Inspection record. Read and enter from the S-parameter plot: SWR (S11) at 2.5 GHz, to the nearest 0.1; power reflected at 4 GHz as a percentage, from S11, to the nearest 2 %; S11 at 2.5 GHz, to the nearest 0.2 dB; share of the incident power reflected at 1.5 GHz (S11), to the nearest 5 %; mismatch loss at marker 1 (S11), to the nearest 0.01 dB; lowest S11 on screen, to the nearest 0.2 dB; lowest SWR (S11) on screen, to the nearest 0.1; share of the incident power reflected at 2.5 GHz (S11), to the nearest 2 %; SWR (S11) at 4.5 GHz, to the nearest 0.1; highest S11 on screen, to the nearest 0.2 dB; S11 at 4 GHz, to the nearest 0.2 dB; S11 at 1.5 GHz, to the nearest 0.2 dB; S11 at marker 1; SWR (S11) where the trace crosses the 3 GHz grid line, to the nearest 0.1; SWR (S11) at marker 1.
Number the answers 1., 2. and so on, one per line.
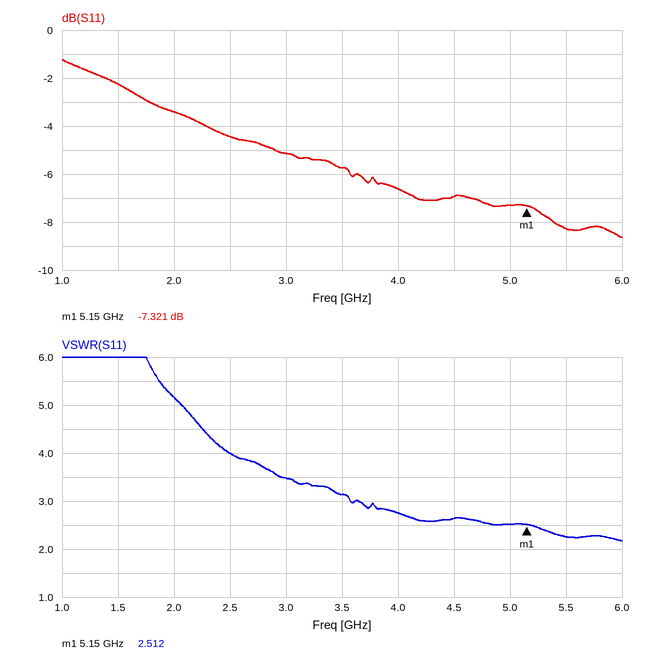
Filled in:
1. 4.0
2. 22 %
3. -4.4 dB
4. 60 %
5. 0.89 dB
6. -8.6 dB
7. 2.2
8. 36 %
9. 2.6
10. -1.2 dB
11. -6.6 dB
12. -2.2 dB
13. -7.321 dB
14. 3.5
15. 2.512
